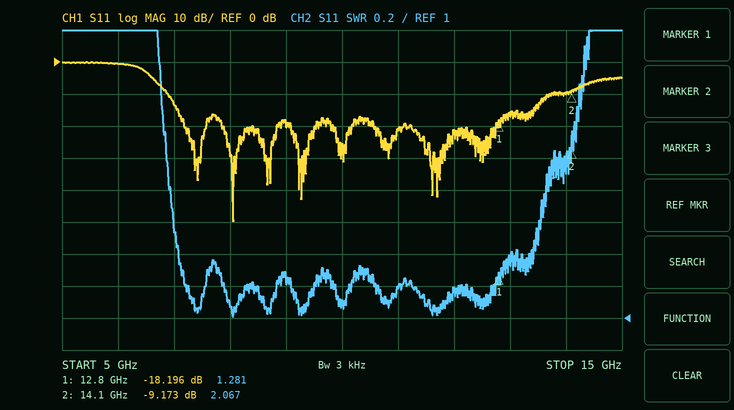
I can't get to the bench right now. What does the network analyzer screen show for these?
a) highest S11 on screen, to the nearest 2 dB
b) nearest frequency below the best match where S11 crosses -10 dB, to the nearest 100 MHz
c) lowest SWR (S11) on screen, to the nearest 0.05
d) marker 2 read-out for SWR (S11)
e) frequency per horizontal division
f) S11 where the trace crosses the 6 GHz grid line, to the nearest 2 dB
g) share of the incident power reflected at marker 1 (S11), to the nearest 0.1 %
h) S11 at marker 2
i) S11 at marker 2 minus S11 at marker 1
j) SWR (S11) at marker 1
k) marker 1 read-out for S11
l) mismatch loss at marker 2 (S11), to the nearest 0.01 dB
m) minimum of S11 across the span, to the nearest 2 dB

0 dB
6.9 GHz
1.00
2.067
1 GHz
0 dB
1.5 %
-9.173 dB
9.023 dB
1.281
-18.196 dB
0.56 dB
-50 dB
